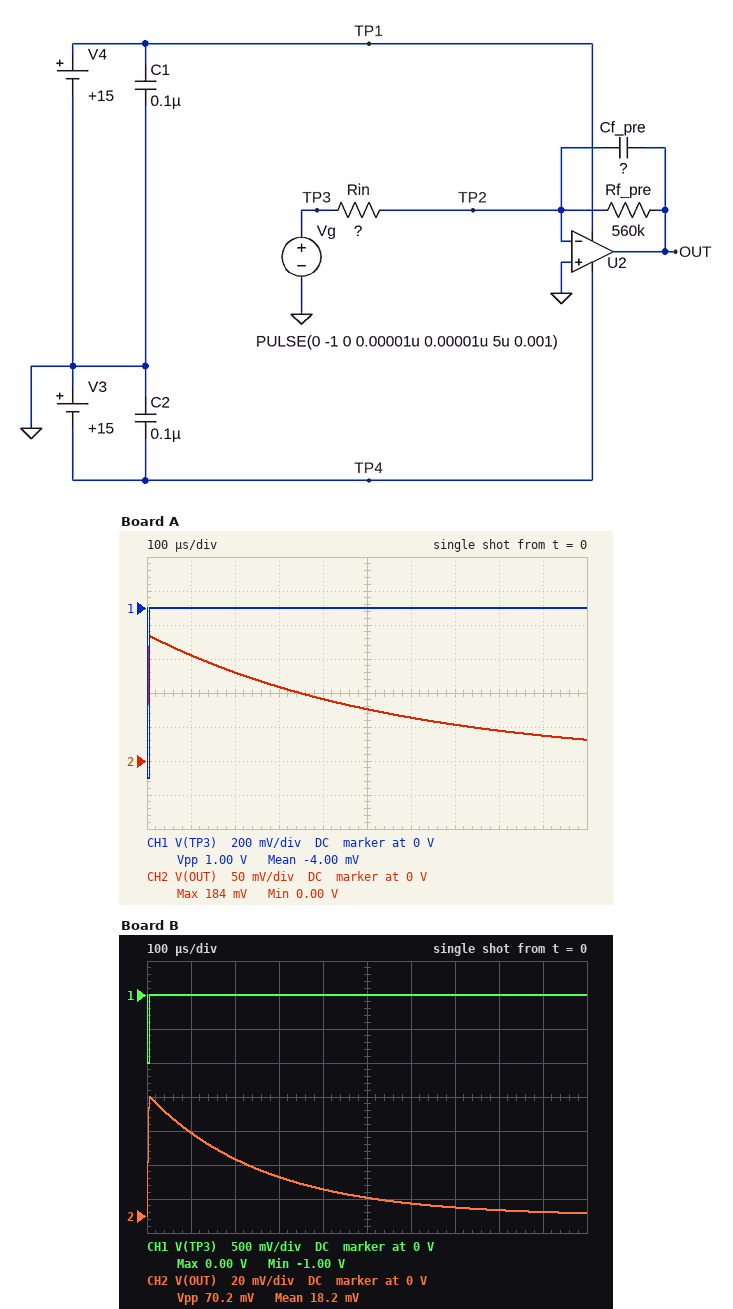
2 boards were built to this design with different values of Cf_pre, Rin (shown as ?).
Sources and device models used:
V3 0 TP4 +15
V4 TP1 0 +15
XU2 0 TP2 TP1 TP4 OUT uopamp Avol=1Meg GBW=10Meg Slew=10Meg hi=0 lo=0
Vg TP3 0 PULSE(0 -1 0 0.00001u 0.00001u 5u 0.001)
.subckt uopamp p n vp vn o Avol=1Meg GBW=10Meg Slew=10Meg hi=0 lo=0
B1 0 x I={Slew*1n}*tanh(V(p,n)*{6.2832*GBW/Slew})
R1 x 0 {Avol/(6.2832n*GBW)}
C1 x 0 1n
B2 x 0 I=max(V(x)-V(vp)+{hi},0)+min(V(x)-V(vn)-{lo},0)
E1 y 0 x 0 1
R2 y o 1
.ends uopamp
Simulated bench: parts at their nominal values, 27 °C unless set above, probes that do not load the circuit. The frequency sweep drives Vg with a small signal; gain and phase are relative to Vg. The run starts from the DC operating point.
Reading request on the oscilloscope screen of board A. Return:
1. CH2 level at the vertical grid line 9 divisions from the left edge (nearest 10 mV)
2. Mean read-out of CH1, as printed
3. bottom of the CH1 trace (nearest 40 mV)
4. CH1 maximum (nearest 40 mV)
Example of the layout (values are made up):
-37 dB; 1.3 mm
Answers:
40 mV; -4.00 mV; -1.00 V; 0 V
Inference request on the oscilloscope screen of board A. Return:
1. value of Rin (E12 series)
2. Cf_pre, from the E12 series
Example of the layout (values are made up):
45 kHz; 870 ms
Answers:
27 kΩ; 1 nF
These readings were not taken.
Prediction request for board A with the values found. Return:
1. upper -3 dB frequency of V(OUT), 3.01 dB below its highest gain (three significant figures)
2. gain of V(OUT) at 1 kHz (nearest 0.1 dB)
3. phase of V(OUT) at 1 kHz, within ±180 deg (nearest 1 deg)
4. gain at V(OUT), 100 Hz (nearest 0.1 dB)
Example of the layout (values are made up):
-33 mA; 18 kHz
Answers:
284 Hz; 15.1 dB; 106 deg; 25.8 dB
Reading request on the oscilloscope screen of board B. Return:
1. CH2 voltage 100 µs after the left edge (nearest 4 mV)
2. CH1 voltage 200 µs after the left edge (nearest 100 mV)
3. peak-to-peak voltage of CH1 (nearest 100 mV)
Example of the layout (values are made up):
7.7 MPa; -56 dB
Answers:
48 mV; 0 V; 1.0 V
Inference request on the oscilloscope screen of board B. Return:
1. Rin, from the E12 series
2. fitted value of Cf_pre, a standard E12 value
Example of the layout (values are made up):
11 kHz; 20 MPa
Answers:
150 kΩ; 470 pF
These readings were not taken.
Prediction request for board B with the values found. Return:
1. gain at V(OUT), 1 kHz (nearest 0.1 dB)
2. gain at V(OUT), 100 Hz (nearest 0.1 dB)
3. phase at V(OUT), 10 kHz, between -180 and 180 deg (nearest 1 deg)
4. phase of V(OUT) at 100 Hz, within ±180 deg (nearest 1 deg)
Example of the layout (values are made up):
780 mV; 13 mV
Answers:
5.7 dB; 11.3 dB; 93 deg; 171 deg
